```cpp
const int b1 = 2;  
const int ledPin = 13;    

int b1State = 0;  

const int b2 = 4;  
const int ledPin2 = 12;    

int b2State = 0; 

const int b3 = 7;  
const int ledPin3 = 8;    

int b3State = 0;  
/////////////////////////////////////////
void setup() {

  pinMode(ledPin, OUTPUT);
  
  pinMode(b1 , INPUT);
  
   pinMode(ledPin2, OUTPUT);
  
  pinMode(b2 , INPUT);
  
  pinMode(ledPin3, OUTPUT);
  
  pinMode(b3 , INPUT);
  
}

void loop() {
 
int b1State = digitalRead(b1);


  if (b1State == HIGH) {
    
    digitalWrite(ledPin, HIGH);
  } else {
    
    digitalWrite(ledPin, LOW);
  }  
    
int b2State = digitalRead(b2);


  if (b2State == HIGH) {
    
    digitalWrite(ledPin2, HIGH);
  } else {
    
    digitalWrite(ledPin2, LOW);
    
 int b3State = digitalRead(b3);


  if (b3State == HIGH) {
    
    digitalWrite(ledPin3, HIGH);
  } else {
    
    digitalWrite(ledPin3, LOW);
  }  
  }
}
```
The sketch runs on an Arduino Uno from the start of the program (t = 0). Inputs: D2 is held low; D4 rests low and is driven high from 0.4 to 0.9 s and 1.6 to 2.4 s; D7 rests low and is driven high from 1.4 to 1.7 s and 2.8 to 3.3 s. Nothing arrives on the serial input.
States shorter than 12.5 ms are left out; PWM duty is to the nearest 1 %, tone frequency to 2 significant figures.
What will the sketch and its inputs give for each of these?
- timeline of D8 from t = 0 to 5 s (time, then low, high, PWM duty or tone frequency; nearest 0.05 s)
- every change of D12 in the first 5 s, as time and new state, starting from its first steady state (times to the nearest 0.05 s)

0 s low; 1.4 s high; 2.4 s low; 2.8 s high; 3.3 s low
0 s low; 0.4 s high; 0.9 s low; 1.6 s high; 2.4 s low
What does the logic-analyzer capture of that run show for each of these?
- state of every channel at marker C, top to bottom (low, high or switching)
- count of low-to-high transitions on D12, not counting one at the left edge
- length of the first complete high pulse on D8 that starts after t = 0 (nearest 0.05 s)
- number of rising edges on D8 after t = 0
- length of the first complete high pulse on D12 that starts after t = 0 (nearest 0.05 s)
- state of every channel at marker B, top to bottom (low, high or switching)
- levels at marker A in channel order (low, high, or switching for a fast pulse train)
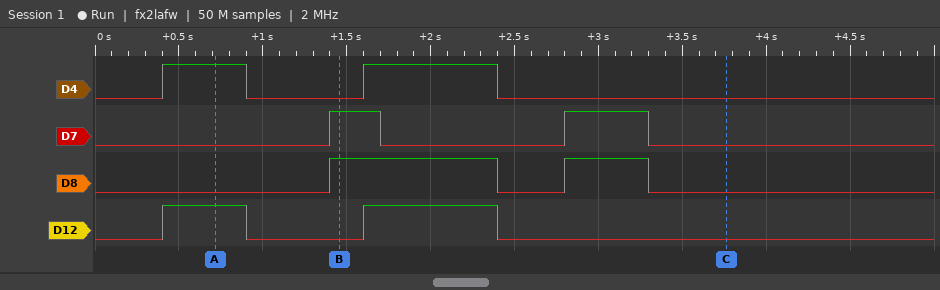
D4 low, D7 low, D8 low, D12 low
2
1.00 s
2
0.50 s
D4 low, D7 high, D8 high, D12 low
D4 high, D7 low, D8 low, D12 high
